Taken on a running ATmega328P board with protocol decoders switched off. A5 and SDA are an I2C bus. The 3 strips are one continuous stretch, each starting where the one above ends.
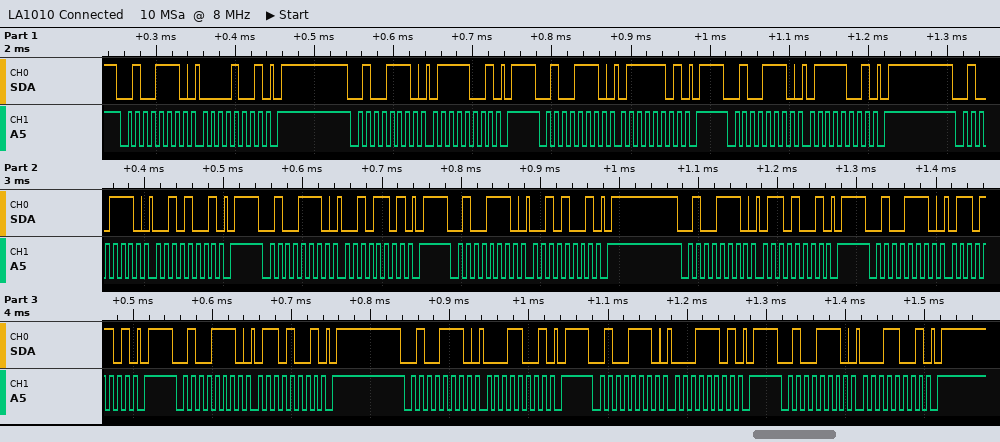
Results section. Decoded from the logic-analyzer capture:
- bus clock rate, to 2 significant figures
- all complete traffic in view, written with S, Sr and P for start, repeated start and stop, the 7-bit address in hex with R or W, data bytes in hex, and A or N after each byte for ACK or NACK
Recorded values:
100 kHz
S 27W A 09 A P S 27W A 79 A P S 27W A 7D A P S 27W A 79 A P S 27W A 29 A P S 27W A 2D A P S 27W A 29 A P S 27W A 69 A P S 27W A 6D A P S 27W A 69 A P S 27W A 19 A P S 27W A 1D A P S 27W A 19 A P
